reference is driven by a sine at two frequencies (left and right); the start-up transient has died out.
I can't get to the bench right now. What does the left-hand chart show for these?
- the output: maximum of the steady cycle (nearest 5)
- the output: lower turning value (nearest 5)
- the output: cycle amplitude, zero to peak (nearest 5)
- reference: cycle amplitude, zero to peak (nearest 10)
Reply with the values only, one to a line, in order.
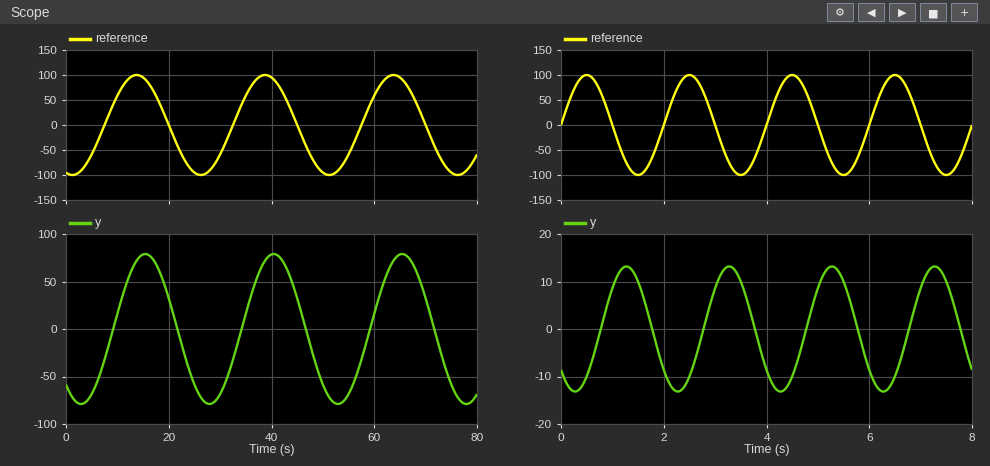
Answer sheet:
80
-80
80
100
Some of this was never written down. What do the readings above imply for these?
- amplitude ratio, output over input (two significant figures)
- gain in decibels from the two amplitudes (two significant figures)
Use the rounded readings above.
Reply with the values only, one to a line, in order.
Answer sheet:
0.80
-1.9 dB
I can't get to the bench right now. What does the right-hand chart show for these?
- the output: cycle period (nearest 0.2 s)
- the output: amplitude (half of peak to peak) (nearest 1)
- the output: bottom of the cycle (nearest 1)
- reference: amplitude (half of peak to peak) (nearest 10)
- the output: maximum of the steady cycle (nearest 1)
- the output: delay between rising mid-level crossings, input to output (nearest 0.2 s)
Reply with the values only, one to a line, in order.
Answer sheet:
2.0 s
13
-13
100
13
0.8 s
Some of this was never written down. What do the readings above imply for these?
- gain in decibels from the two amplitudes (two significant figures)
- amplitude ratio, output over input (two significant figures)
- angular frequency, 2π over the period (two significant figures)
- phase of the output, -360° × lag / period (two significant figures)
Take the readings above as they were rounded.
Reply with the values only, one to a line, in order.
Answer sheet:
-18 dB
0.13
3.1 rad/s
-140°
